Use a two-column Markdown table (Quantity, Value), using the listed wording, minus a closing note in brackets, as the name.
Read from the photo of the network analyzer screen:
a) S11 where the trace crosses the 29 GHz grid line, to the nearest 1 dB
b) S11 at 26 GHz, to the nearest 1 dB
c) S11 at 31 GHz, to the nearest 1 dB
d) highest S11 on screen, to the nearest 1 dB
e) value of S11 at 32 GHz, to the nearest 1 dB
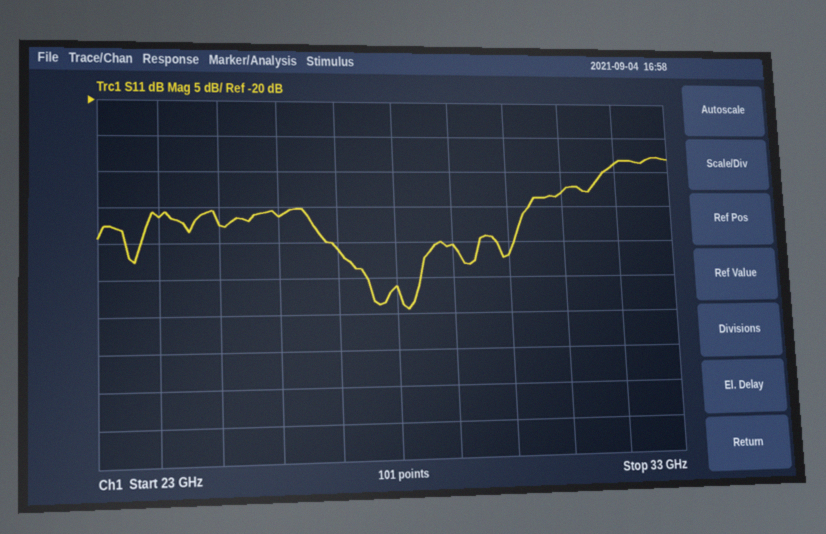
| Quantity | Value |
|---|---|
| S11 where the trace crosses the 29 GHz grid line, to the nearest 1 dB | -40 dB |
| S11 at 26 GHz, to the nearest 1 dB | -36 dB |
| S11 at 31 GHz, to the nearest 1 dB | -33 dB |
| highest S11 on screen, to the nearest 1 dB | -28 dB |
| value of S11 at 32 GHz, to the nearest 1 dB | -29 dB |
